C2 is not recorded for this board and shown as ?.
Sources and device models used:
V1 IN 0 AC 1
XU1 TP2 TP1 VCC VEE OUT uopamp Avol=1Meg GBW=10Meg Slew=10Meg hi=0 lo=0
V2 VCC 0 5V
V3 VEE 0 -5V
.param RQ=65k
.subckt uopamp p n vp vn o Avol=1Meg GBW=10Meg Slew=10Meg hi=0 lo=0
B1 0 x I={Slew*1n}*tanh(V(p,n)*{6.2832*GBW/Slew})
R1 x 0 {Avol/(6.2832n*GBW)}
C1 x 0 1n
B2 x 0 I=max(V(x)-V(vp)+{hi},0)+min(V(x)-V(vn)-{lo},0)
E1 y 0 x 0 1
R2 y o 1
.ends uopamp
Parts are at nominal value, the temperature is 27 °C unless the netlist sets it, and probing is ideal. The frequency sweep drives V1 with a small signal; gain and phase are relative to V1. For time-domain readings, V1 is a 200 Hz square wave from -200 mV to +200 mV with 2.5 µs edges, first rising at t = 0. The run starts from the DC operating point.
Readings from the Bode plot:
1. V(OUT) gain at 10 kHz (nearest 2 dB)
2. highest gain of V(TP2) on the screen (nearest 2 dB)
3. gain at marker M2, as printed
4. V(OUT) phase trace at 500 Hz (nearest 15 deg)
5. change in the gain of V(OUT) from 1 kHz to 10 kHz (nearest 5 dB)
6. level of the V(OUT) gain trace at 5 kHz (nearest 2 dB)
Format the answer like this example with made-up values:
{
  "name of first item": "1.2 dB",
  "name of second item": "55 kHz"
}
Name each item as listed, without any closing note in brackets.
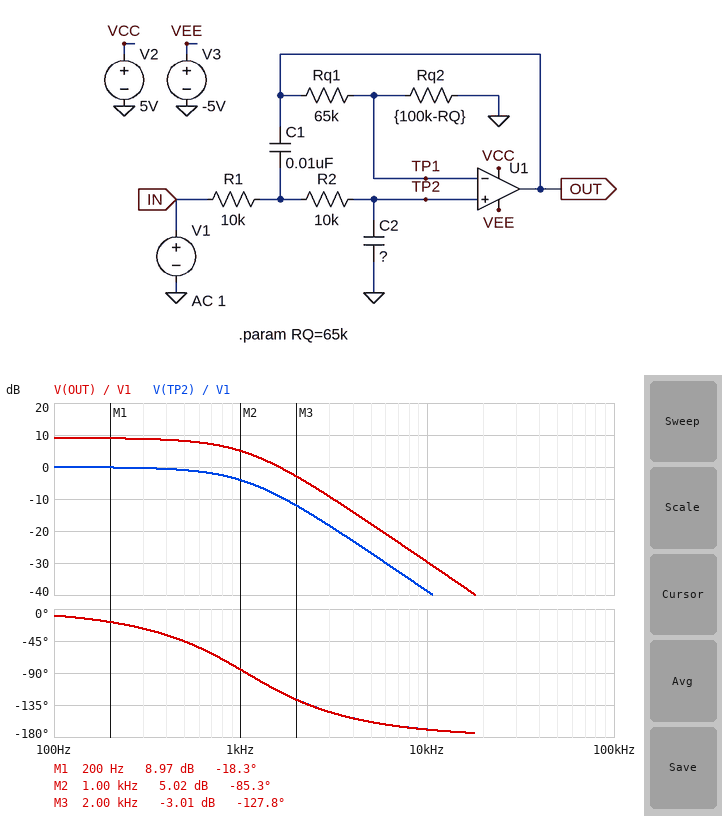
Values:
{
  "V(OUT) gain at 10 kHz": "-30 dB",
  "highest gain of V(TP2) on the screen": "0 dB",
  "gain at marker M2, as printed": "5.02 dB",
  "V(OUT) phase trace at 500 Hz": "-45 deg",
  "change in the gain of V(OUT) from 1 kHz to 10 kHz": "-35 dB",
  "level of the V(OUT) gain trace at 5 kHz": "-18 dB"
}
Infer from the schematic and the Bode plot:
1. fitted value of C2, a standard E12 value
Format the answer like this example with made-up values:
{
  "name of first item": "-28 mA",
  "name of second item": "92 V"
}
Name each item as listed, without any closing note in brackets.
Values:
{
  "fitted value of C2, a standard E12 value": "22 nF"
}
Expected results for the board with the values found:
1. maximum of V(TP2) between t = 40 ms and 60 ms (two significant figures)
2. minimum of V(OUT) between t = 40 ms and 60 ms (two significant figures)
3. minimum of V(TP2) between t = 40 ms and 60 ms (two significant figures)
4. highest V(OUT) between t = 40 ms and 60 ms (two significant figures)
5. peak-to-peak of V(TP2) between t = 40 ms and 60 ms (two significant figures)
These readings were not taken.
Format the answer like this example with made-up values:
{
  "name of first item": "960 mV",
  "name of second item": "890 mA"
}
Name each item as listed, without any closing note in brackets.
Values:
{
  "maximum of V(TP2) between t = 40 ms and 60 ms": "200 mV",
  "minimum of V(OUT) between t = 40 ms and 60 ms": "-580 mV",
  "minimum of V(TP2) between t = 40 ms and 60 ms": "-200 mV",
  "highest V(OUT) between t = 40 ms and 60 ms": "580 mV",
  "peak-to-peak of V(TP2) between t = 40 ms and 60 ms": "400 mV"
}
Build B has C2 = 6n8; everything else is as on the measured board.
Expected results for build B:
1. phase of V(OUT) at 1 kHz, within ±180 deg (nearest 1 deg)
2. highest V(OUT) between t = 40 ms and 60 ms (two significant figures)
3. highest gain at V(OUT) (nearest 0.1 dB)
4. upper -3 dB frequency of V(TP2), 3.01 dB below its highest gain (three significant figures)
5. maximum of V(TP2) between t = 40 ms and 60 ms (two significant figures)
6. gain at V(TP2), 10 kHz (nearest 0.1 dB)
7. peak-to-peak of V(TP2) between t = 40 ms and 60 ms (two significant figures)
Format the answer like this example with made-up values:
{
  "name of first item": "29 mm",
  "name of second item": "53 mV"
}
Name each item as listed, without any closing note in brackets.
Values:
{
  "phase of V(OUT) at 1 kHz, within ±180 deg": "23 deg",
  "highest V(OUT) between t = 40 ms and 60 ms": "5.0 V",
  "highest gain at V(OUT)": "13.9 dB",
  "upper -3 dB frequency of V(TP2), 3.01 dB below its highest gain": "2.28 kHz",
  "maximum of V(TP2) between t = 40 ms and 60 ms": "2.6 V",
  "gain at V(TP2), 10 kHz": "-28.3 dB",
  "peak-to-peak of V(TP2) between t = 40 ms and 60 ms": "5.2 V"
}
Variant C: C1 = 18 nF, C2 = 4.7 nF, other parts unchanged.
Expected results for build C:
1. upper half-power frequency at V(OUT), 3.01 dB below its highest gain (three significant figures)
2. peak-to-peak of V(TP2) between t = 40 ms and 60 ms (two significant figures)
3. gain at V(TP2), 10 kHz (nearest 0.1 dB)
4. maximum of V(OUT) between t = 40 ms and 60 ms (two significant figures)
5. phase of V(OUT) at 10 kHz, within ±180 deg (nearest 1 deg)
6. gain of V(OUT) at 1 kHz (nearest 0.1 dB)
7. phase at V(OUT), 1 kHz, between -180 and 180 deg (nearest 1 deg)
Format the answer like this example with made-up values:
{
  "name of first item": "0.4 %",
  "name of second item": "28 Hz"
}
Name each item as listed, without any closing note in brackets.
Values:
{
  "upper half-power frequency at V(OUT), 3.01 dB below its highest gain": "772 Hz",
  "peak-to-peak of V(TP2) between t = 40 ms and 60 ms": "8.9 V",
  "gain at V(TP2), 10 kHz": "-31.1 dB",
  "maximum of V(OUT) between t = 40 ms and 60 ms": "5.0 V",
  "phase of V(OUT) at 10 kHz, within ±180 deg": "155 deg",
  "gain of V(OUT) at 1 kHz": "4.8 dB",
  "phase at V(OUT), 1 kHz, between -180 and 180 deg": "66 deg"
}
